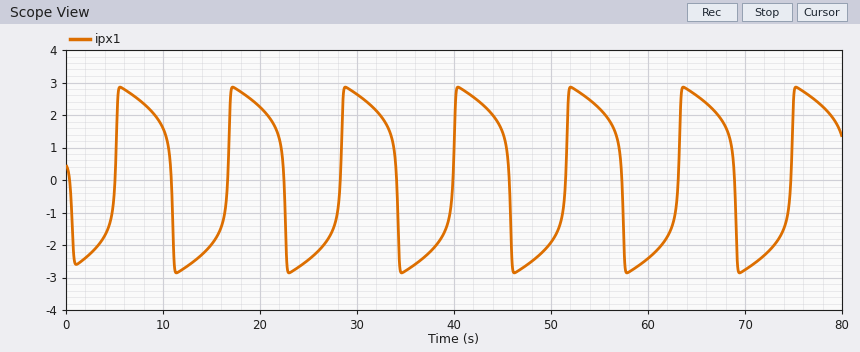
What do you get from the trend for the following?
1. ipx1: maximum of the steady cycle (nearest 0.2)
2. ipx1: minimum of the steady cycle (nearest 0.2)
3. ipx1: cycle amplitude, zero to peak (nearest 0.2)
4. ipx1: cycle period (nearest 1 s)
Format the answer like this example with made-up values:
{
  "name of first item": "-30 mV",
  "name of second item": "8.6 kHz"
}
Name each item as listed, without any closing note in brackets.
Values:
{
  "ipx1: maximum of the steady cycle": "2.8",
  "ipx1: minimum of the steady cycle": "-2.8",
  "ipx1: cycle amplitude, zero to peak": "2.8",
  "ipx1: cycle period": "12 s"
}
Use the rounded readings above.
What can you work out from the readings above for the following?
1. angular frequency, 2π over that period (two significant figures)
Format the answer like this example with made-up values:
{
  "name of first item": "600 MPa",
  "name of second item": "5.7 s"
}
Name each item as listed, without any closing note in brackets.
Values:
{
  "angular frequency, 2π over that period": "0.52 rad/s"
}
